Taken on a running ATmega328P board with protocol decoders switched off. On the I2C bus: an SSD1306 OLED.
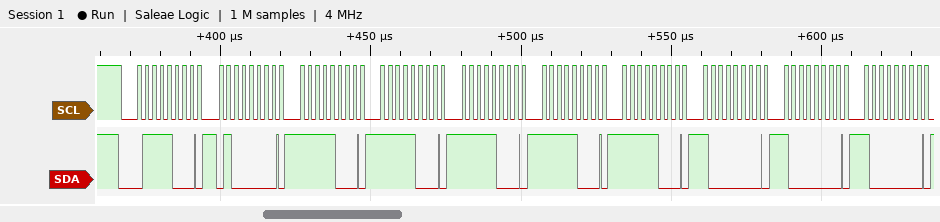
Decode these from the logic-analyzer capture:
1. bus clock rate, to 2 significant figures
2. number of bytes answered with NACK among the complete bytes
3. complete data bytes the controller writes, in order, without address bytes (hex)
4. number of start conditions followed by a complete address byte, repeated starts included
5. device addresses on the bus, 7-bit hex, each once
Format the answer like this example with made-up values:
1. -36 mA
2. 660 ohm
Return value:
1. 400 kHz
2. 0
3. 40 F8 F8 F8 F8 F8 80 80 80
4. 1
5. 0x3C
